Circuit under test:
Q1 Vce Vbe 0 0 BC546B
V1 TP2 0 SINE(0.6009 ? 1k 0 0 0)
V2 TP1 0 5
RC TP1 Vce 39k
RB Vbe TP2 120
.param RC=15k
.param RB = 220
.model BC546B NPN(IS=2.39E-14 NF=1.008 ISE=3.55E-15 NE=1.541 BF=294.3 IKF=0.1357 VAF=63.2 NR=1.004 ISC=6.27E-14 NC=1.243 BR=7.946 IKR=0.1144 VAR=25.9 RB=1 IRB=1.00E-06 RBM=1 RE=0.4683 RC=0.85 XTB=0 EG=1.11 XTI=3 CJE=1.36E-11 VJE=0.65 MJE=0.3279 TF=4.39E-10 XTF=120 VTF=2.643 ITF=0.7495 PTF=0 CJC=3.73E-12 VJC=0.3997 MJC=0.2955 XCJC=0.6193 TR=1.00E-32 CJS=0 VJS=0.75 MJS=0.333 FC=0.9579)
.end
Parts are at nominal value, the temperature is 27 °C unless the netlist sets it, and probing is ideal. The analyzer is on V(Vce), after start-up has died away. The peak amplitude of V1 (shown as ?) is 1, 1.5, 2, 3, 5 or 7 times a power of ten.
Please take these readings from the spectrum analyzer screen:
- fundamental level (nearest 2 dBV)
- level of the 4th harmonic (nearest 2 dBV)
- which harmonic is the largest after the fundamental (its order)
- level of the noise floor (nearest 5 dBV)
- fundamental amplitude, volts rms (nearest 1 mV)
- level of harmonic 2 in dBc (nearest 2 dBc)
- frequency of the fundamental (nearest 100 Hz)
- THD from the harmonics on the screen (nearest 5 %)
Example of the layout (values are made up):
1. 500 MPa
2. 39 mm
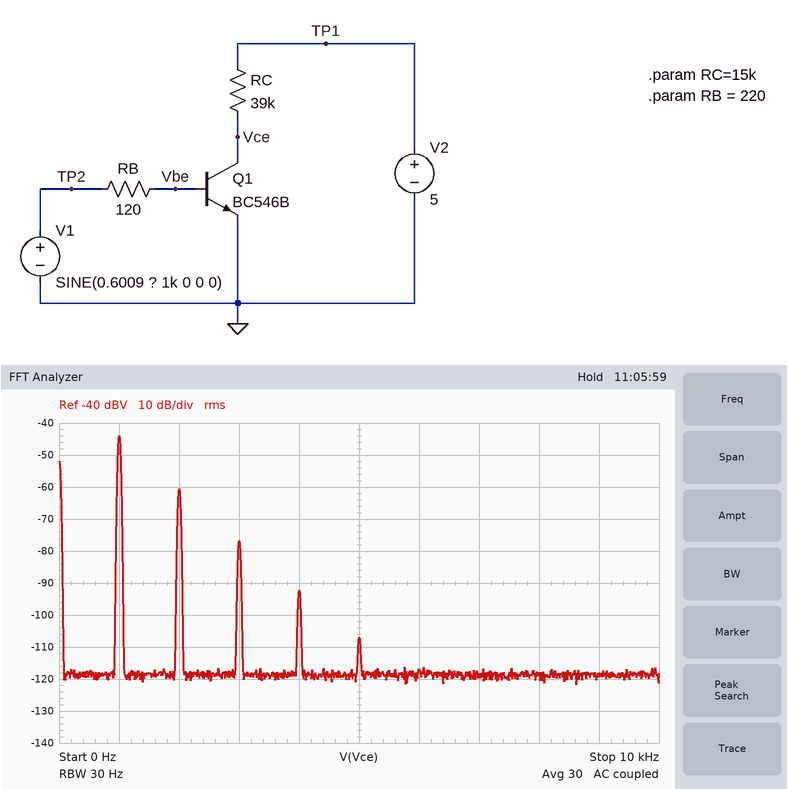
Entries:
1. -44 dBV
2. -92 dBV
3. 2
4. -120 dBV
5. 6 mV
6. -16 dBc
7. 1.0 kHz
8. 15 %
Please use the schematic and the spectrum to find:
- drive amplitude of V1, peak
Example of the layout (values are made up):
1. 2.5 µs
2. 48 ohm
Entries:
1. 7 mV
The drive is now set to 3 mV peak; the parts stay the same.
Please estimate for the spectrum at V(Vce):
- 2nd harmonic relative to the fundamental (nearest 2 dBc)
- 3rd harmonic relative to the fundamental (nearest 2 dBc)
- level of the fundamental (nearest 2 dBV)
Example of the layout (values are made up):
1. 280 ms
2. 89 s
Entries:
1. -24 dBc
2. -48 dBc
3. -52 dBV
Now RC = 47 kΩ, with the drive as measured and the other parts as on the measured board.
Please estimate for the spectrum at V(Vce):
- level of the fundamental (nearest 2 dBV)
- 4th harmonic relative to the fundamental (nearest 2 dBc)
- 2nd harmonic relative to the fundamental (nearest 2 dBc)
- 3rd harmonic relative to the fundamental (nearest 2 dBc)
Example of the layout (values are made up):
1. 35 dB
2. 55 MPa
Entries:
1. -48 dBV
2. -54 dBc
3. -18 dBc
4. -36 dBc
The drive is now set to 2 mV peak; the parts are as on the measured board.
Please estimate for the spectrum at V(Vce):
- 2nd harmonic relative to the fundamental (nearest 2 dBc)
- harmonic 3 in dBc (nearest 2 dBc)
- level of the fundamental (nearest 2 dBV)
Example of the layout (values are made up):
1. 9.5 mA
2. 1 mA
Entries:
1. -28 dBc
2. -56 dBc
3. -56 dBV
